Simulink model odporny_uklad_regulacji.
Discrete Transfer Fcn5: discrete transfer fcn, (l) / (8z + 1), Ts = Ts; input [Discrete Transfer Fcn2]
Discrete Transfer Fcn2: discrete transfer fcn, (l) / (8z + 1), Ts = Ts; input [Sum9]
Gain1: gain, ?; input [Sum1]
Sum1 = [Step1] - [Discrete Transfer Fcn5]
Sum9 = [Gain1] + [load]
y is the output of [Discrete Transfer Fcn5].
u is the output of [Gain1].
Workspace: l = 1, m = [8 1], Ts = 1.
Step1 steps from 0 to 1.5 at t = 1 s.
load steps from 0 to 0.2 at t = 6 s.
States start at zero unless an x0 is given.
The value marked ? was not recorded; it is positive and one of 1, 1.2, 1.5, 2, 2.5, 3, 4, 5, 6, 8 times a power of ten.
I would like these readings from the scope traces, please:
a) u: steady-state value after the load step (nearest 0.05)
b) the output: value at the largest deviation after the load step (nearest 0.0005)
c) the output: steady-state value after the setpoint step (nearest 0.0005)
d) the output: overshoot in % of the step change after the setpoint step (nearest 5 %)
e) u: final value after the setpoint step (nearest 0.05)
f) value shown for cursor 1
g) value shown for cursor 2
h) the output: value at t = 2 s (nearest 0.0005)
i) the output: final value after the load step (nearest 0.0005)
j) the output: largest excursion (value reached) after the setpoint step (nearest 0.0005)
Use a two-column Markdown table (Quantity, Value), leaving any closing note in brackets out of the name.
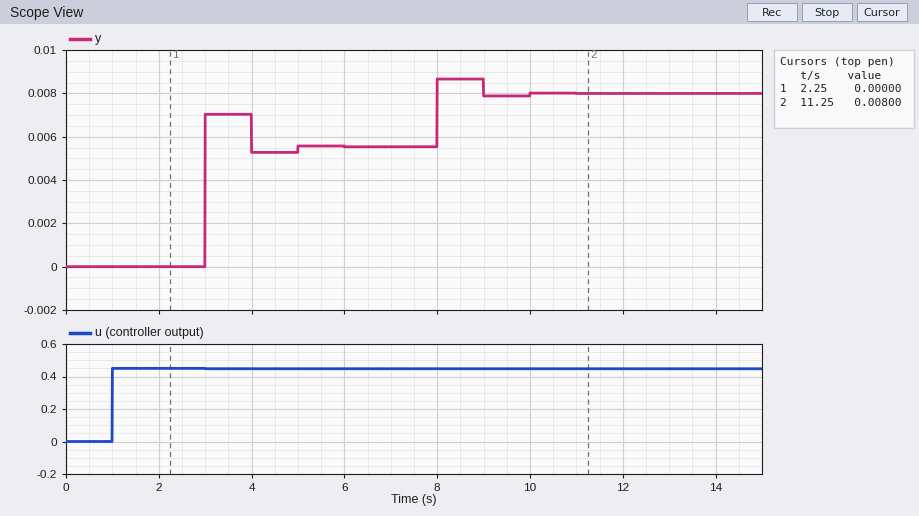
| Quantity | Value |
|---|---|
| u: steady-state value after the load step | 0.45 |
| the output: value at the largest deviation after the load step | 0.0085 |
| the output: steady-state value after the setpoint step | 0.0055 |
| the output: overshoot in % of the step change after the setpoint step | 25 % |
| u: final value after the setpoint step | 0.45 |
| value shown for cursor 1 | 0.00000 |
| value shown for cursor 2 | 0.00800 |
| the output: value at t = 2 s | 0.0000 |
| the output: final value after the load step | 0.0080 |
| the output: largest excursion (value reached) after the setpoint step | 0.0070 |
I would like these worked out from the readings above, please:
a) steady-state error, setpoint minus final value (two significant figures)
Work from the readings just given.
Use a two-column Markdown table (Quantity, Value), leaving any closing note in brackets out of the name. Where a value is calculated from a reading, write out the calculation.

| Quantity | Value |
|---|---|
| steady-state error, setpoint minus final value | 1.5 - 0.0055 = 1.5 |
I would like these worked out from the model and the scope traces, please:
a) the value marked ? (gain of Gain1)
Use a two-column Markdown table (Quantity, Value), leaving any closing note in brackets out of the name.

| Quantity | Value |
|---|---|
| the value marked ? | 0.3 |
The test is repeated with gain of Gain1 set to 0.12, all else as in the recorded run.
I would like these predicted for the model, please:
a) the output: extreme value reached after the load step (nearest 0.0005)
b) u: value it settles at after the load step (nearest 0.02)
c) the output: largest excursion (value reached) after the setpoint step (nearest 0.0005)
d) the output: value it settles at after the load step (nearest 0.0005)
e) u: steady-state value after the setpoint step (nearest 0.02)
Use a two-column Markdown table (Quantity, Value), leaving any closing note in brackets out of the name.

| Quantity | Value |
|---|---|
| the output: extreme value reached after the load step | 0.0055 |
| u: value it settles at after the load step | 0.18 |
| the output: largest excursion (value reached) after the setpoint step | 0.0030 |
| the output: value it settles at after the load step | 0.0045 |
| u: steady-state value after the setpoint step | 0.18 |
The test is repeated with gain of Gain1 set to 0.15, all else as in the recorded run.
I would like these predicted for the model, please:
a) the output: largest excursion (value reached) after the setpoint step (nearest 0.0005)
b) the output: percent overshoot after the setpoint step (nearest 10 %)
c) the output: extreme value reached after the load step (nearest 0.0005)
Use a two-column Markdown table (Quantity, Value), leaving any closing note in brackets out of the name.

| Quantity | Value |
|---|---|
| the output: largest excursion (value reached) after the setpoint step | 0.0035 |
| the output: percent overshoot after the setpoint step | 30 % |
| the output: extreme value reached after the load step | 0.0060 |
